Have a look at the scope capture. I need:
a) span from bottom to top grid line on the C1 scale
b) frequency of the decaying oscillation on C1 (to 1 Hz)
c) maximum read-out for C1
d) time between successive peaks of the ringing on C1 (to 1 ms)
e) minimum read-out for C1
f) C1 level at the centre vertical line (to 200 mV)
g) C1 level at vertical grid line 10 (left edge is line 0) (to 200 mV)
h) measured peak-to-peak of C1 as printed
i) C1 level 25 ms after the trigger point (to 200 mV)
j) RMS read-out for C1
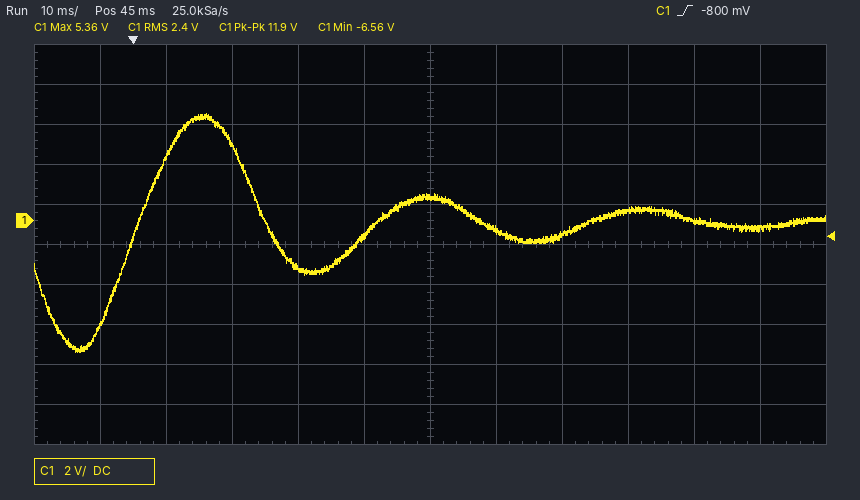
20 V
30 Hz
5.36 V
33 ms
-6.56 V
1.2 V
0.0 V
11.9 V
-2.4 V
2.4 V
